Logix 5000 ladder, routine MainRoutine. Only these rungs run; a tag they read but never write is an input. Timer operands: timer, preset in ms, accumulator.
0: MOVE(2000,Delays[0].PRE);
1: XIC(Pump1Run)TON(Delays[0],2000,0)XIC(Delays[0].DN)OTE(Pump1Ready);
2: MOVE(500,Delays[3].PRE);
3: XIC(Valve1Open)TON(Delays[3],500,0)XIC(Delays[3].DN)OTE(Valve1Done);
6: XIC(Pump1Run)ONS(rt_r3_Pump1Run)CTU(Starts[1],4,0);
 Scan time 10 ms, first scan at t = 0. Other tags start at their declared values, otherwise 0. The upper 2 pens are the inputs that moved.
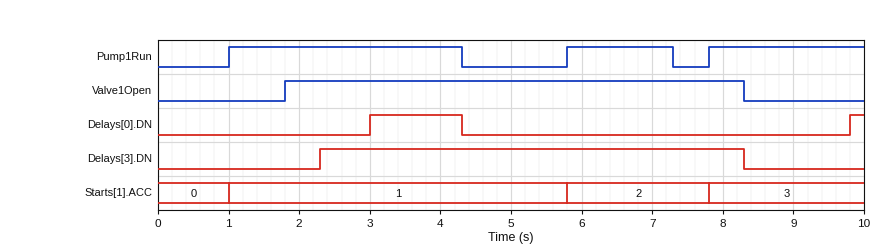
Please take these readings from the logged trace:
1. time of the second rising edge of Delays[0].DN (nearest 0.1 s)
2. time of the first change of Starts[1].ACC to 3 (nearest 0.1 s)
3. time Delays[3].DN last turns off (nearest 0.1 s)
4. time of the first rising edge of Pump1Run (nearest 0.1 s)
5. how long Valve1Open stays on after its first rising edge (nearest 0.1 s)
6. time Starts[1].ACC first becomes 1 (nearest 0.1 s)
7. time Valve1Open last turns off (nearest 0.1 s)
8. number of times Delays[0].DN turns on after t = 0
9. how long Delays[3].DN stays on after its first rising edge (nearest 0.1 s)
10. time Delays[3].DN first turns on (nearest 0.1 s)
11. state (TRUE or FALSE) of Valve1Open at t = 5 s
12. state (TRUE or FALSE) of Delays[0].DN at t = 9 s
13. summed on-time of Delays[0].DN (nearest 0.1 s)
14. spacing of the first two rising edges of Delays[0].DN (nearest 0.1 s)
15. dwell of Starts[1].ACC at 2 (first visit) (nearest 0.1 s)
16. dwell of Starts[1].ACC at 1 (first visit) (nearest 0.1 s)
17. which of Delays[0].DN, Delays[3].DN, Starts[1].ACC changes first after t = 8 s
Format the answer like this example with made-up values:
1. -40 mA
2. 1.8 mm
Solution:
1. 9.8 s
2. 7.8 s
3. 8.3 s
4. 1.0 s
5. 6.5 s
6. 1.0 s
7. 8.3 s
8. 2
9. 6.0 s
10. 2.3 s
11. TRUE
12. FALSE
13. 1.5 s
14. 6.8 s
15. 2.0 s
16. 4.8 s
17. Delays[3].DN
